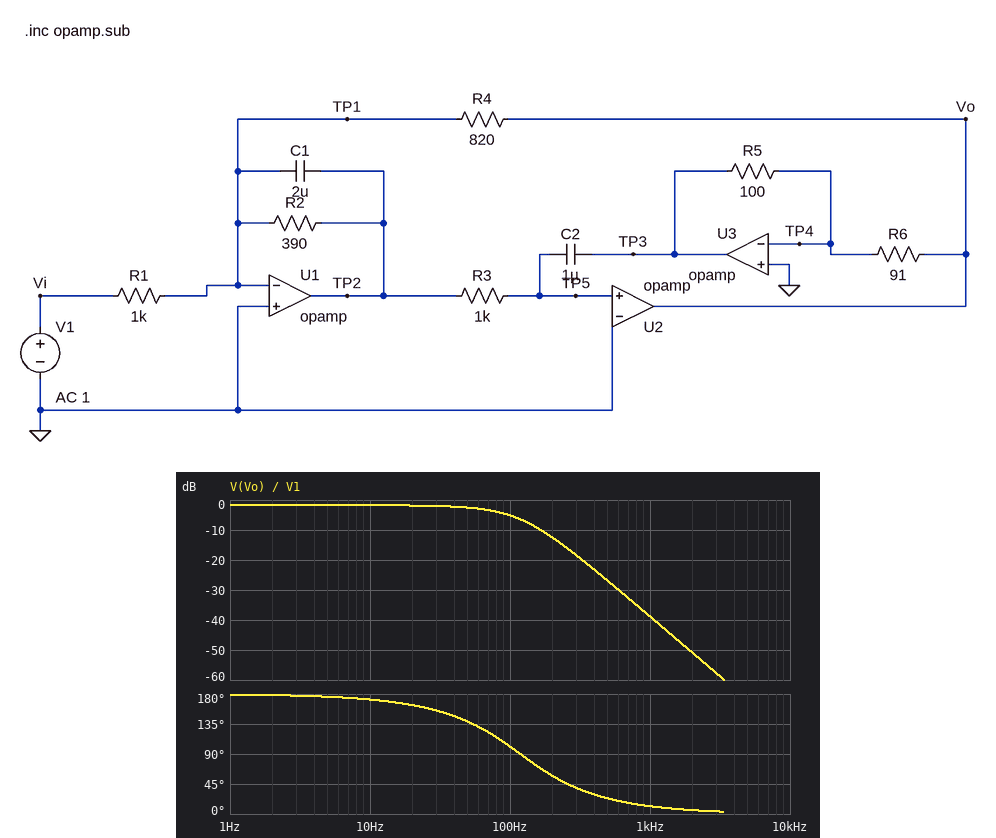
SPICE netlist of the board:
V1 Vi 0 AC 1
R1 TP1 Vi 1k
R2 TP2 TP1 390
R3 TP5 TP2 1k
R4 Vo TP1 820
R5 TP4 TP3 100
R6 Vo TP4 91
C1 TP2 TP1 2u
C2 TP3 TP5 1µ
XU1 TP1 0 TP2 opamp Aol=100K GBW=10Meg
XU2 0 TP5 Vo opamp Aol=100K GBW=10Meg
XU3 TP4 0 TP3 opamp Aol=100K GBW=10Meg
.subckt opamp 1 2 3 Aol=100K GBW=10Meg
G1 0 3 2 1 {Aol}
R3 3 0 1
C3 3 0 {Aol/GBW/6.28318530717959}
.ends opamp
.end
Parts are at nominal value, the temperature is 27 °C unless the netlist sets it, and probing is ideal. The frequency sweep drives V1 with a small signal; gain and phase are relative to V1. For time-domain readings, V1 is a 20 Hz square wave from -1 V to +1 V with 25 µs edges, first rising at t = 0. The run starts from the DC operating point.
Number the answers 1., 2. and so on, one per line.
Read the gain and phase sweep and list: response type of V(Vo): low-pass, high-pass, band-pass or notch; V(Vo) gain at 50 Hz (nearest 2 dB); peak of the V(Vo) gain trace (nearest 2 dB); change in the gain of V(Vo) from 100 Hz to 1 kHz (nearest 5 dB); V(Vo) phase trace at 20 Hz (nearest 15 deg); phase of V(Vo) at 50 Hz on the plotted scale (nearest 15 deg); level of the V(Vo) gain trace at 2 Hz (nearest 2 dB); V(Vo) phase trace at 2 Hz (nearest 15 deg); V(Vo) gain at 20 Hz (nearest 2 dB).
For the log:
1. low-pass
2. -2 dB
3. -2 dB
4. -35 dB
5. 165 deg
6. 135 deg
7. -2 dB
8. 180 deg
9. -2 dB
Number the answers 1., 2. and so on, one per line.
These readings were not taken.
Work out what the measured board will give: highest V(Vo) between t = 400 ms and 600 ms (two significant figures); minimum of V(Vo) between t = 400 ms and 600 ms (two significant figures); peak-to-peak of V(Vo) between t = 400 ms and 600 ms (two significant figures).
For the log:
1. 830 mV
2. -830 mV
3. 1.7 V
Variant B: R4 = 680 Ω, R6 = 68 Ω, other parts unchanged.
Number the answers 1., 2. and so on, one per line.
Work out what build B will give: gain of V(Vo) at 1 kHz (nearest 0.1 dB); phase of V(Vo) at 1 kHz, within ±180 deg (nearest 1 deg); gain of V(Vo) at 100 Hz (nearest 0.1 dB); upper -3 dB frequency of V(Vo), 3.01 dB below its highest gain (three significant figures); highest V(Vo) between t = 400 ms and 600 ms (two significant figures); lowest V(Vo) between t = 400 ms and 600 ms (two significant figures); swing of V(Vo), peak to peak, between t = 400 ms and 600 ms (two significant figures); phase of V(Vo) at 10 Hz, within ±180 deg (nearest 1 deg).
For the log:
1. -41.4 dB
2. 12 deg
3. -7.6 dB
4. 83.1 Hz
5. 680 mV
6. -680 mV
7. 1.4 V
8. 171 deg
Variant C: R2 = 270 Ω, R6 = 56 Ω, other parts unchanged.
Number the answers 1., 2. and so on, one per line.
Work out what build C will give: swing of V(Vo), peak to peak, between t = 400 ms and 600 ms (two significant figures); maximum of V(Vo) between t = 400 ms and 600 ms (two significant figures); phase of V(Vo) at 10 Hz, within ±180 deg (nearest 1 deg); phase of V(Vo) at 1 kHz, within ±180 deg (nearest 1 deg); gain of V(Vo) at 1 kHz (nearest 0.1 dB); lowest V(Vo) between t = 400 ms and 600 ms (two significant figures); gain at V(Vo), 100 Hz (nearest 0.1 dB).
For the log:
1. 1.6 V
2. 810 mV
3. 161 deg
4. 17 deg
5. -43.3 dB
6. -810 mV
7. -12.4 dB
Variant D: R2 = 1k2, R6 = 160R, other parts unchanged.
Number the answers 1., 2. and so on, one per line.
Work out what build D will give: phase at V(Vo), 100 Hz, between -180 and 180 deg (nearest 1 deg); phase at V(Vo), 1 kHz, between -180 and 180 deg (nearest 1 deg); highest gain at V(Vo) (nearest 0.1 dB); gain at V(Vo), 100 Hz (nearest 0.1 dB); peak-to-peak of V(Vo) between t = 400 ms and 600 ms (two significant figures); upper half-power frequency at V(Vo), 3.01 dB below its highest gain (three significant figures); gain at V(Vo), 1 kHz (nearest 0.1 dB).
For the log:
1. 156 deg
2. 4 deg
3. 6.0 dB
4. 2.0 dB
5. 3.3 V
6. 181 Hz
7. -33.7 dB
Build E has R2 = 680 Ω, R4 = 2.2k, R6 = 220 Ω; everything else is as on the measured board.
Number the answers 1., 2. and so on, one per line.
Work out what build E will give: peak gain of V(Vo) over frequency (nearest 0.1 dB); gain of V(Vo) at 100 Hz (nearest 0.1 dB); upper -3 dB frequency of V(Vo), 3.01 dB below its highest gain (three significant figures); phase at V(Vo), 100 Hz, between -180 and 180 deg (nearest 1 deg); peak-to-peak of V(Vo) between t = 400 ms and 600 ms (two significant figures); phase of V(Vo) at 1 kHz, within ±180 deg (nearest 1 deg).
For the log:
1. 7.9 dB
2. 7.3 dB
3. 131 Hz
4. 103 deg
5. 5.7 V
6. 7 deg
